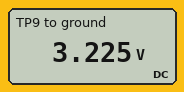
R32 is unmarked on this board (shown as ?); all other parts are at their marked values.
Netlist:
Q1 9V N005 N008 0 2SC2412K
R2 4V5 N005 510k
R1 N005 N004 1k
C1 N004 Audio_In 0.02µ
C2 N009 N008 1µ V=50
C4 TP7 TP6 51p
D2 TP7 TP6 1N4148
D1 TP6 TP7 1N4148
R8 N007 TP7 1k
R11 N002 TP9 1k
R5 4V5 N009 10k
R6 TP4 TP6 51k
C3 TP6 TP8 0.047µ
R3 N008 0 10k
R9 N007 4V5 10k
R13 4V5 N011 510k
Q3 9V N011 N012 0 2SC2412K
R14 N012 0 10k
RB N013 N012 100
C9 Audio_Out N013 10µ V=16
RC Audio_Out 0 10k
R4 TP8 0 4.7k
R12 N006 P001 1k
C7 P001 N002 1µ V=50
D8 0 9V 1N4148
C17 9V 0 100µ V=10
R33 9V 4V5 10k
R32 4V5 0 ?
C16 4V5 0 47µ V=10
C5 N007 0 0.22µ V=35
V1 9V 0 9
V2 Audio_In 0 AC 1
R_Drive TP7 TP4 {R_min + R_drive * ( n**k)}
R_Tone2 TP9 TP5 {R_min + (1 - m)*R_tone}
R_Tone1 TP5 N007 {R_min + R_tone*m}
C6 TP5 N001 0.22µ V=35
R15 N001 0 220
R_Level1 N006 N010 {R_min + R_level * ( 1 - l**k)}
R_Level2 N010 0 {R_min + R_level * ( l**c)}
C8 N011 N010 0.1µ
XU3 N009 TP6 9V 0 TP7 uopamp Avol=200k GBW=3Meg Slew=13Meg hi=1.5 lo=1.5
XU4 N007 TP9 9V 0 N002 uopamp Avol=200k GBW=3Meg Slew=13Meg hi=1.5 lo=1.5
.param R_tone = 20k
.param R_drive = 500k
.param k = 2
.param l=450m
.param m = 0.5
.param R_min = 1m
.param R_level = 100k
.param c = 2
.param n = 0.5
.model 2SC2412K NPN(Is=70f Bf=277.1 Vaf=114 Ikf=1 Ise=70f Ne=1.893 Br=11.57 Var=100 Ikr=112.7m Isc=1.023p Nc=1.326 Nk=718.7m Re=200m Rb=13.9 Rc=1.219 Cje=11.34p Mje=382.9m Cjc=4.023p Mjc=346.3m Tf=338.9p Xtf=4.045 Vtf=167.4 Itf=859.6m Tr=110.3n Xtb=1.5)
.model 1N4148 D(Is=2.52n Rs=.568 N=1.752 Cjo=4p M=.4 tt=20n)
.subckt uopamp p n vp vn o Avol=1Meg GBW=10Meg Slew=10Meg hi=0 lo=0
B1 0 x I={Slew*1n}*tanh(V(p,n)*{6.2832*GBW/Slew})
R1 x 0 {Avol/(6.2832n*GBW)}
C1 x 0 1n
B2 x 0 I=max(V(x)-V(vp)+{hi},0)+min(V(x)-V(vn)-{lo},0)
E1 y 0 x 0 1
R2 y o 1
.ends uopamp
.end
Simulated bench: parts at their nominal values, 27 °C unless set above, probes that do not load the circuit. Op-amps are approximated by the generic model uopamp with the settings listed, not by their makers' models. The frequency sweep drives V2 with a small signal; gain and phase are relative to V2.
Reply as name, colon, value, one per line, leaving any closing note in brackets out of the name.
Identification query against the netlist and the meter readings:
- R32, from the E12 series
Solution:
R32, from the E12 series: 5.6 kΩ
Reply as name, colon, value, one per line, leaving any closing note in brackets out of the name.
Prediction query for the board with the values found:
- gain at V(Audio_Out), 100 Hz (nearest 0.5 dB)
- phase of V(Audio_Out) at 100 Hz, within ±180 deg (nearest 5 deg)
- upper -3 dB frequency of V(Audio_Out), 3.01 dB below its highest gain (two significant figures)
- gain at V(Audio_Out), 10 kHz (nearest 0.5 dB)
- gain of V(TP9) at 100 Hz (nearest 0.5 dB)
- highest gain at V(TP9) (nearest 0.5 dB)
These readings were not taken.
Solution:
gain at V(Audio_Out), 100 Hz: -1.5 dB
phase of V(Audio_Out) at 100 Hz, within ±180 deg: 90 deg
upper -3 dB frequency of V(Audio_Out), 3.01 dB below its highest gain: 1.9 kHz
gain at V(Audio_Out), 10 kHz: -7.5 dB
gain of V(TP9) at 100 Hz: 12.5 dB
highest gain at V(TP9): 24.5 dB
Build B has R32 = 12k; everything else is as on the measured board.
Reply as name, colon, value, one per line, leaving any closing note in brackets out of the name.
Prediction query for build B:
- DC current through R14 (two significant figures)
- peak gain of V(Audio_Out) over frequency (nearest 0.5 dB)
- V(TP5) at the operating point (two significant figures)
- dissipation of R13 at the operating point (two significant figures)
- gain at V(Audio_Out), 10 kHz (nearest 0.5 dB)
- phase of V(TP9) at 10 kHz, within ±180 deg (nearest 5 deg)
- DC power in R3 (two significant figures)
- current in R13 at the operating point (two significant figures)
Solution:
DC current through R14: 370 µA
peak gain of V(Audio_Out) over frequency: 11.0 dB
V(TP5) at the operating point: 4.9 V
dissipation of R13 at the operating point: 840 nW
gain at V(Audio_Out), 10 kHz: -7.0 dB
phase of V(TP9) at 10 kHz, within ±180 deg: -120 deg
DC power in R3: 1.3 mW
current in R13 at the operating point: 1.3 µA
